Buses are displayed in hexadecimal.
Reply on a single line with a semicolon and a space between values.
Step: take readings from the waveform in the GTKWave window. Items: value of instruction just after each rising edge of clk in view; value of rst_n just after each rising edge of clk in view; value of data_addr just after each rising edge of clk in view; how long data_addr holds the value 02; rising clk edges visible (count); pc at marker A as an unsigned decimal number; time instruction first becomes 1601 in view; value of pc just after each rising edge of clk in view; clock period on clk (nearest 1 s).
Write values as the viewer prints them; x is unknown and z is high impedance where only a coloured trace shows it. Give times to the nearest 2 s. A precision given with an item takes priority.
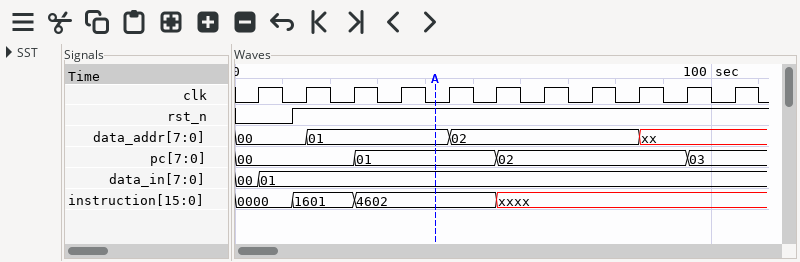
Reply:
0000, 1601, 4602, 4602, 4602, xxxx, xxxx, xxxx, xxxx, xxxx, xxxx; 0 1 1 1 1 1 1 1 1 1 1; 00, 01, 01, 01, 02, 02, 02, 02, xx, xx, xx; 40 s; 11; 1; 12 s; 00, 00, 01, 01, 01, 02, 02, 02, 02, 03, 03; 10 s
